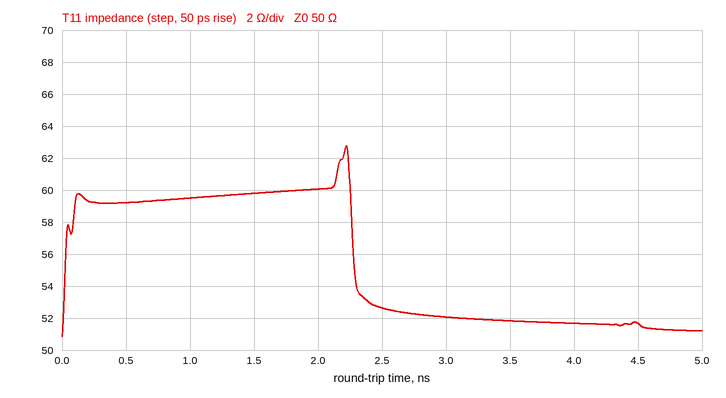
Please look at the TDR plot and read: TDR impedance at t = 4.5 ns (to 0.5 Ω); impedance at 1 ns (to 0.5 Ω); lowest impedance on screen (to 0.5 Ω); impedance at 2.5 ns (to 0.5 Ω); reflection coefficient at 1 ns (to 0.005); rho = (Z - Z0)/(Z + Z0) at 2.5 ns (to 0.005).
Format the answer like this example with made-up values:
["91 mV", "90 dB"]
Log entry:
["51.5 Ω", "59.5 Ω", "51.0 Ω", "52.5 Ω", "+0.085", "+0.025"]
